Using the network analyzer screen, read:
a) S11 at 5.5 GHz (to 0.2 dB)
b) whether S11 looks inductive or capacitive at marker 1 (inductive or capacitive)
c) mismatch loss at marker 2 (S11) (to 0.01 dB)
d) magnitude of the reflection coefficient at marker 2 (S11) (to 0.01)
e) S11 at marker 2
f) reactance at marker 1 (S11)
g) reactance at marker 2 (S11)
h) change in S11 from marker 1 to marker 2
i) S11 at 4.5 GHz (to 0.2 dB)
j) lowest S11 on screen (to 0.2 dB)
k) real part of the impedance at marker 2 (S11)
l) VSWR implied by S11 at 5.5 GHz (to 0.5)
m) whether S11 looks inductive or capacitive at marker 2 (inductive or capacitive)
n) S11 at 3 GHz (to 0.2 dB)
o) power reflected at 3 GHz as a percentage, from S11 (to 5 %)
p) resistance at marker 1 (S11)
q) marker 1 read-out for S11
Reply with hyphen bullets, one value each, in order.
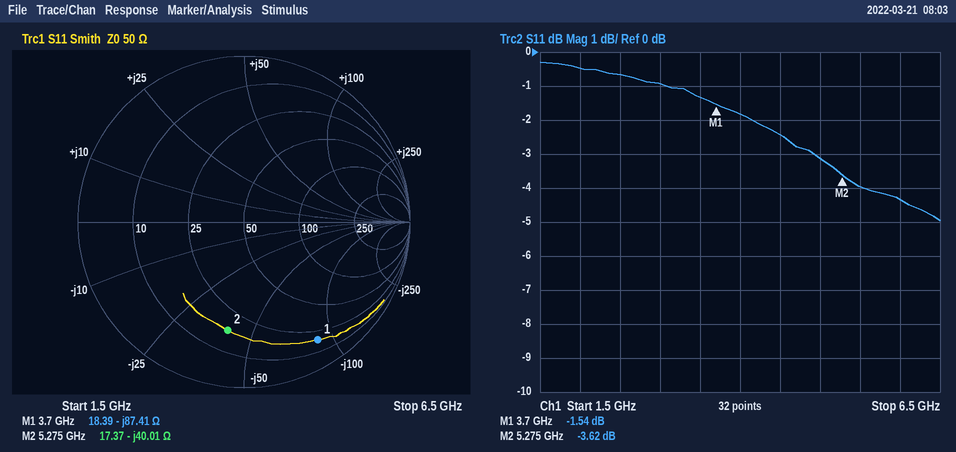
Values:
- -4.0 dB
- capacitive
- 2.48 dB
- 0.66
- -3.62 dB
- -87.41 Ω
- -40.01 Ω
- -2.08 dB
- -2.4 dB
- -5.0 dB
- 17.37 Ω
- 4.5
- capacitive
- -1.0 dB
- 80 %
- 18.39 Ω
- -1.54 dB
